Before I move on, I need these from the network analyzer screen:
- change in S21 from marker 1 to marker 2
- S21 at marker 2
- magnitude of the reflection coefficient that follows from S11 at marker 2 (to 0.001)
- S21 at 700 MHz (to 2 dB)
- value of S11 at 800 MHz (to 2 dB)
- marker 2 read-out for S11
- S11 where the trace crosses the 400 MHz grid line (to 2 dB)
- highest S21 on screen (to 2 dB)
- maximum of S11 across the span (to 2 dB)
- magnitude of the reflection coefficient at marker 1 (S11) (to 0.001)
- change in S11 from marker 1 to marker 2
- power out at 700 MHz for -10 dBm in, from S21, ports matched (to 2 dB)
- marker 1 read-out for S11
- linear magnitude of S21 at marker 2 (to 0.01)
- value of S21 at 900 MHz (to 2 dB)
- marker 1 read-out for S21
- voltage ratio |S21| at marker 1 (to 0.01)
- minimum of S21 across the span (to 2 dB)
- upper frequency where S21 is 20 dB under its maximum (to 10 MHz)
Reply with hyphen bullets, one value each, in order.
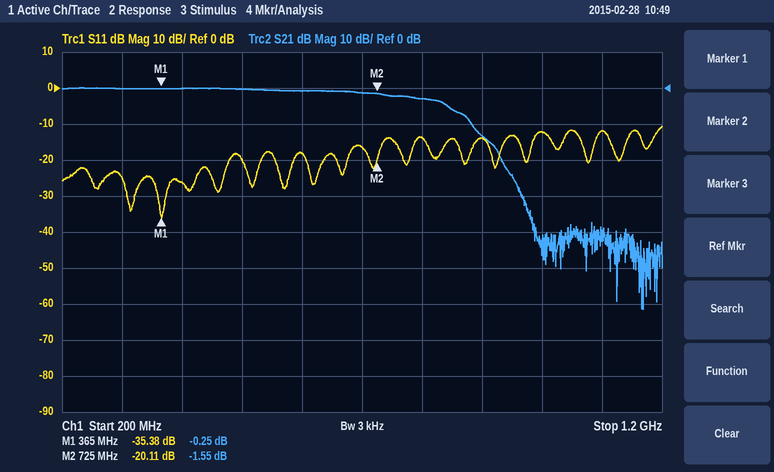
- -1.30 dB
- -1.55 dB
- 0.099
- -2 dB
- -14 dB
- -20.11 dB
- -26 dB
- 0 dB
- -10 dB
- 0.017
- 15.27 dB
- -12 dBm
- -35.38 dB
- 0.84
- -14 dB
- -0.25 dB
- 0.97
- -62 dB
- 930 MHz
